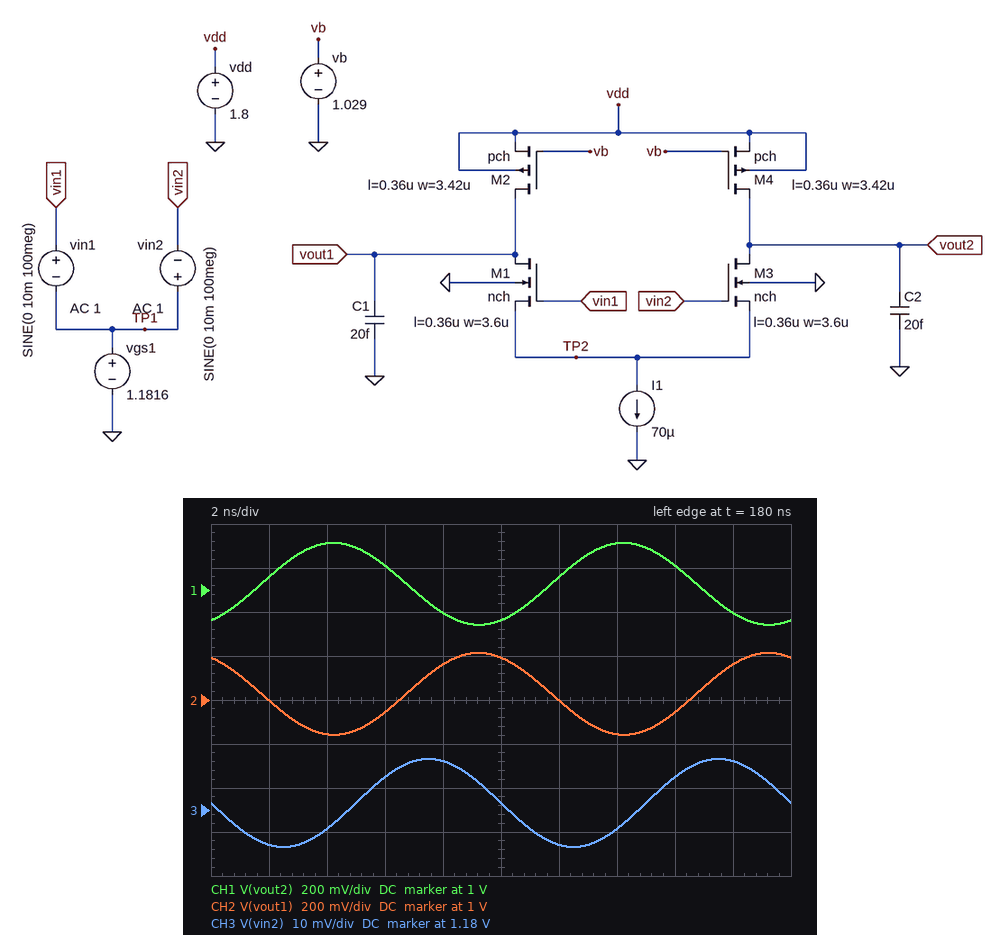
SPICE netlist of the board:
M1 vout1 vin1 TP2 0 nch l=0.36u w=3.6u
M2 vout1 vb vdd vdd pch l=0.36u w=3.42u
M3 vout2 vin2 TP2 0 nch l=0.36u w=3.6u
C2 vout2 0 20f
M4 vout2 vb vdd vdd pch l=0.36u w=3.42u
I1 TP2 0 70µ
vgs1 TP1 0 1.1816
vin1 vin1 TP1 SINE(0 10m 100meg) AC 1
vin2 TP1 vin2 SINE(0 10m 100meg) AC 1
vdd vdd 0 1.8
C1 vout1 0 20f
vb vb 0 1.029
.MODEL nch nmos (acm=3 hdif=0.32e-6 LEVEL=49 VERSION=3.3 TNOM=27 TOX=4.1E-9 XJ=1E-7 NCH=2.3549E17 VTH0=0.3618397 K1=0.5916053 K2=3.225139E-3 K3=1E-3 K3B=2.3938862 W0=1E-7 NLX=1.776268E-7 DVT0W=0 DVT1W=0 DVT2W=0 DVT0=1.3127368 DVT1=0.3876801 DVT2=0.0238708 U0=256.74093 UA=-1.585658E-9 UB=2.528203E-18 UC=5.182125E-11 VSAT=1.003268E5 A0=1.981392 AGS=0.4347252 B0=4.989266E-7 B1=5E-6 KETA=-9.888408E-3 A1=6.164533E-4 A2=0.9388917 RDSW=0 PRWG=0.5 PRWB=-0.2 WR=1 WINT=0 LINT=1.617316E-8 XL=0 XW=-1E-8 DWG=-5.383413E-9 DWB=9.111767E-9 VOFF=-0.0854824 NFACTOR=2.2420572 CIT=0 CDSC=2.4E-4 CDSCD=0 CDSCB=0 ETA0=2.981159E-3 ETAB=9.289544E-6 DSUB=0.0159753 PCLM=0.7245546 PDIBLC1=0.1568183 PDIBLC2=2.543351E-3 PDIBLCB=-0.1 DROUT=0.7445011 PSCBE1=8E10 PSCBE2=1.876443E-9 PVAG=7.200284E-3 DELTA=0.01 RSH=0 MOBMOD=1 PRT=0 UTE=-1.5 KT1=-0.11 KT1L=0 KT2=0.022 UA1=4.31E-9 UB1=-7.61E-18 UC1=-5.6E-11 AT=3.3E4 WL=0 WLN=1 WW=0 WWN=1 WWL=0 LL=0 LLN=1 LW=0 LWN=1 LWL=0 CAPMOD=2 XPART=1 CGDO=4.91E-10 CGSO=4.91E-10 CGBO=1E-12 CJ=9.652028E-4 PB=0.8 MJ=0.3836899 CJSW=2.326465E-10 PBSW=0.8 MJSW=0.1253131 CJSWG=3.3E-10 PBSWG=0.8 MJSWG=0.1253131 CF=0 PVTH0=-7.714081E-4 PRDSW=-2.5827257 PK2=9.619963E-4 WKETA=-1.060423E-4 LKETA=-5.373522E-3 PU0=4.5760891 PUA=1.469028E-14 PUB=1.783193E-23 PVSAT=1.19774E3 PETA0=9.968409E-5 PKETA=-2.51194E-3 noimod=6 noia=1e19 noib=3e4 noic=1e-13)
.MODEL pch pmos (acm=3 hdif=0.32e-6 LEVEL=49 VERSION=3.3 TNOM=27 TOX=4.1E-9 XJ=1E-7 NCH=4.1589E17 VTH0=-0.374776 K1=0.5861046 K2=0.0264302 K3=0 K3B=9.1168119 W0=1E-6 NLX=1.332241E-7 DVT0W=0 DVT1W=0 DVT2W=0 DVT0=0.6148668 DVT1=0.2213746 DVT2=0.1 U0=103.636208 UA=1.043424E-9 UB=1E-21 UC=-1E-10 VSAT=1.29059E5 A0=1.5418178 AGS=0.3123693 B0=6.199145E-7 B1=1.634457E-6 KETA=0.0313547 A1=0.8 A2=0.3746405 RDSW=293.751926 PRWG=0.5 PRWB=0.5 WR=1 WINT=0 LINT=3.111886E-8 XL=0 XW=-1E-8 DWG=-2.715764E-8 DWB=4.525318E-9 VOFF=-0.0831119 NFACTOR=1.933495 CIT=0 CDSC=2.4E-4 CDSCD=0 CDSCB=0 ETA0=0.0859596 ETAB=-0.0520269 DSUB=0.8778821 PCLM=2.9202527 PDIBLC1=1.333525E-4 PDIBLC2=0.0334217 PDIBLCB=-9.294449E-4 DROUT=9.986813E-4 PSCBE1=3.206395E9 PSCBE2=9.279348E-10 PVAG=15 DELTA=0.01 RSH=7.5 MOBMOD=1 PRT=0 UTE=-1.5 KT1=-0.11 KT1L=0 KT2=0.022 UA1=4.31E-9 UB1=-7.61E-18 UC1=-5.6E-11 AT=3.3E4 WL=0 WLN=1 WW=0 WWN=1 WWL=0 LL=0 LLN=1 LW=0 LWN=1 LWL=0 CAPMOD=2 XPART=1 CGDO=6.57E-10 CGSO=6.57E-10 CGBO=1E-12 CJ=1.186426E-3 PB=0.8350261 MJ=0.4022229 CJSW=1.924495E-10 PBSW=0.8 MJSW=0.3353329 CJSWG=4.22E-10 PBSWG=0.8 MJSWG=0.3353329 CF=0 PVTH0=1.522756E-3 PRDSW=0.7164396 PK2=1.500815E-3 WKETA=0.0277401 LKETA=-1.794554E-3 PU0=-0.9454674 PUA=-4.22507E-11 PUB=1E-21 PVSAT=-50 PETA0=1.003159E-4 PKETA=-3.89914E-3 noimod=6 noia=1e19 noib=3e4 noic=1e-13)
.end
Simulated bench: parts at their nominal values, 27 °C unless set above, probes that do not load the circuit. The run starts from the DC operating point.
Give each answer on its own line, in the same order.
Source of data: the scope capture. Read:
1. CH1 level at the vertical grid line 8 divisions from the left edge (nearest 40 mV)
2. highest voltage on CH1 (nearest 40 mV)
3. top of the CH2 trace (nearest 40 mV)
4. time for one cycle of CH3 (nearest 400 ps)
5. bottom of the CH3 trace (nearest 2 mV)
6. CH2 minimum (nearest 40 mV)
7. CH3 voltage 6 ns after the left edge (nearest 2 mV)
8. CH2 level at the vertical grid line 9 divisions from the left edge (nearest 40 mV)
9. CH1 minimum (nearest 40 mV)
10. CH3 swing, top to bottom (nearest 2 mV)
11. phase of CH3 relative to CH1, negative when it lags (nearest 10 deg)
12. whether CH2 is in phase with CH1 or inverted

1.12 V
1.20 V
1.20 V
10.0 ns
1.172 V
840 mV
1.188 V
1.16 V
840 mV
20 mV
-120 deg
inverted
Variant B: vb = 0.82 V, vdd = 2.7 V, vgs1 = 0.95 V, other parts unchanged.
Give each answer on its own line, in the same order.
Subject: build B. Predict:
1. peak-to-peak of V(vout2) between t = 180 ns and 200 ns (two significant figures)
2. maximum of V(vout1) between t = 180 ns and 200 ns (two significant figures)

11 mV
2.7 V
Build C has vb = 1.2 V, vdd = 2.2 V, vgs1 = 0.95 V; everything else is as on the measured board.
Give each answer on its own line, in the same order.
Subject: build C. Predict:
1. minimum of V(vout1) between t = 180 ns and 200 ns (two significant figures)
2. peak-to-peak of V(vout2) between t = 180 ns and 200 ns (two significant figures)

2.1 V
29 mV
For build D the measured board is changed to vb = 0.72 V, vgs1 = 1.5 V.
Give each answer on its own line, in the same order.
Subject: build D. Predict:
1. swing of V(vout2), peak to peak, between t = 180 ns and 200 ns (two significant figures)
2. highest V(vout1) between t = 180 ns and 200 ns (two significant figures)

24 mV
1.7 V
